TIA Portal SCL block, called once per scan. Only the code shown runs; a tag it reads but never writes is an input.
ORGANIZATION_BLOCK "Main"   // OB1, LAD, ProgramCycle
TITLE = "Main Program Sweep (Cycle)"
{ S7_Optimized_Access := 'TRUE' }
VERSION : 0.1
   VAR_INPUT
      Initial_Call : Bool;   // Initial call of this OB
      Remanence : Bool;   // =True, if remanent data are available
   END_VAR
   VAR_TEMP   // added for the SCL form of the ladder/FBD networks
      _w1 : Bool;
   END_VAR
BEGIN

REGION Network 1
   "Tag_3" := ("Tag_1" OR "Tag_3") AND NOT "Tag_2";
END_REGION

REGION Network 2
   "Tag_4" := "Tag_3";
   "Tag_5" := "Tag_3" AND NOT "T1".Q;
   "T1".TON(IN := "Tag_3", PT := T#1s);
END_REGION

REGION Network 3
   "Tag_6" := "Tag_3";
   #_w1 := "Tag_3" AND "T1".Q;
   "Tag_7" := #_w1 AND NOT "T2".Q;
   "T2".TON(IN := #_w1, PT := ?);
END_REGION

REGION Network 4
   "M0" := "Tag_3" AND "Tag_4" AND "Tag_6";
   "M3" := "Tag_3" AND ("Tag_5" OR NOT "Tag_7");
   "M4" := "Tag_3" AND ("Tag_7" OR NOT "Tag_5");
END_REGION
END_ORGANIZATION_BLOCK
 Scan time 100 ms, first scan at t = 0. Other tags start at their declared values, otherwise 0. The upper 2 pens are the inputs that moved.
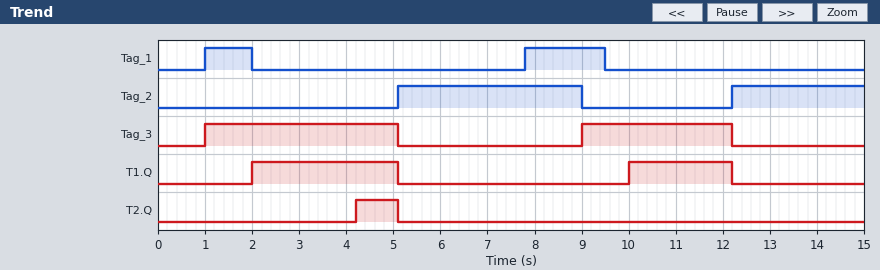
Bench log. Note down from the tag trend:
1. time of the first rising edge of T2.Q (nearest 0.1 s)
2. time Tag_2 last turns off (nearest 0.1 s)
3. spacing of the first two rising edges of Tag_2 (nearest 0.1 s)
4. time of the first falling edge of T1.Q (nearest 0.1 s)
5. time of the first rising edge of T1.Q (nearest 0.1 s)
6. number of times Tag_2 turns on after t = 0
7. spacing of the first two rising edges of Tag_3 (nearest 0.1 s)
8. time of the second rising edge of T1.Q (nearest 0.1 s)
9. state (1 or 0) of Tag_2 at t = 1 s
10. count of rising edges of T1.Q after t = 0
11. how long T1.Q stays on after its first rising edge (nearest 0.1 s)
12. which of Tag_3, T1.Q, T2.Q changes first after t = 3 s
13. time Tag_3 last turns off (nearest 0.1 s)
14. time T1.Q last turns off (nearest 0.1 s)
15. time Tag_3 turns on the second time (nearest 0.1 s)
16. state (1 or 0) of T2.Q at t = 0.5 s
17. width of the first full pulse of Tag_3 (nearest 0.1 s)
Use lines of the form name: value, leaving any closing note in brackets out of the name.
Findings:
time of the first rising edge of T2.Q: 4.2 s
time Tag_2 last turns off: 9.0 s
spacing of the first two rising edges of Tag_2: 7.1 s
time of the first falling edge of T1.Q: 5.1 s
time of the first rising edge of T1.Q: 2.0 s
number of times Tag_2 turns on after t = 0: 2
spacing of the first two rising edges of Tag_3: 8.0 s
time of the second rising edge of T1.Q: 10.0 s
state (1 or 0) of Tag_2 at t = 1 s: 0
count of rising edges of T1.Q after t = 0: 2
how long T1.Q stays on after its first rising edge: 3.1 s
which of Tag_3, T1.Q, T2.Q changes first after t = 3 s: T2.Q
time Tag_3 last turns off: 12.2 s
time T1.Q last turns off: 12.2 s
time Tag_3 turns on the second time: 9.0 s
state (1 or 0) of T2.Q at t = 0.5 s: 0
width of the first full pulse of Tag_3: 4.1 s
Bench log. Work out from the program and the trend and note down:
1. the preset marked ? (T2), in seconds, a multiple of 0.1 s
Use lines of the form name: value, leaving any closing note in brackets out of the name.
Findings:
the preset marked ? (T2), in seconds, a multiple of 0.1 s: 2.2 s
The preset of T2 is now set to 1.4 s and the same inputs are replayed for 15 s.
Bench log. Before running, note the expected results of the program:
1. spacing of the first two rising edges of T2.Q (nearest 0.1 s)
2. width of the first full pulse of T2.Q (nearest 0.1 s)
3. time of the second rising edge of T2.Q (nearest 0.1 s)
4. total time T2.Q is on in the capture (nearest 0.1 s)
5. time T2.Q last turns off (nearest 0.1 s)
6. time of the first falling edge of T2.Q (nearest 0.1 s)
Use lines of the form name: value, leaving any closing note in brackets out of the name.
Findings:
spacing of the first two rising edges of T2.Q: 8.0 s
width of the first full pulse of T2.Q: 1.7 s
time of the second rising edge of T2.Q: 11.4 s
total time T2.Q is on in the capture: 2.5 s
time T2.Q last turns off: 12.2 s
time of the first falling edge of T2.Q: 5.1 s
